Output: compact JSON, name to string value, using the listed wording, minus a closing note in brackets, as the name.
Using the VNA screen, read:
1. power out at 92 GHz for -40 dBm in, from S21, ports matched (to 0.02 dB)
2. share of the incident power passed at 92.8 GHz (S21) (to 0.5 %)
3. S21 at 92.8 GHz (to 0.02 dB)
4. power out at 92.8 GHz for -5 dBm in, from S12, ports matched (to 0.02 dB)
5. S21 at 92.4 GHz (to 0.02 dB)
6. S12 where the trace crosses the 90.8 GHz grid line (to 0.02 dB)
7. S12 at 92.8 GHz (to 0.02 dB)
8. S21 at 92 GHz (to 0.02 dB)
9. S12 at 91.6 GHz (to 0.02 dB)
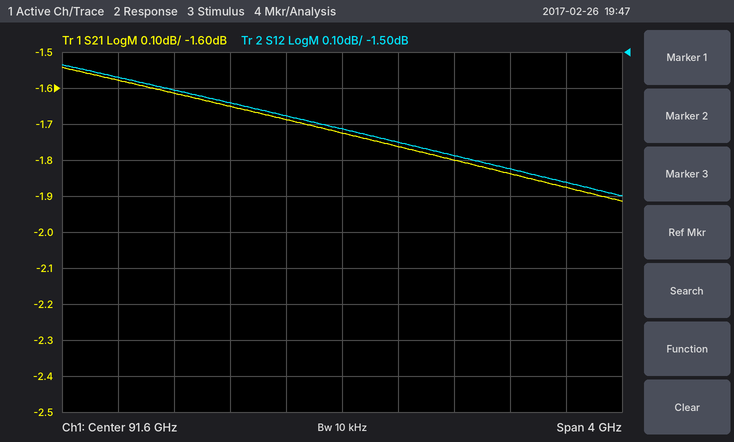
{"power out at 92 GHz for -40 dBm in, from S21, ports matched": "-41.76 dBm", "share of the incident power passed at 92.8 GHz (S21)": "65.5 %", "S21 at 92.8 GHz": "-1.84 dB", "power out at 92.8 GHz for -5 dBm in, from S12, ports matched": "-6.82 dBm", "S21 at 92.4 GHz": "-1.80 dB", "S12 where the trace crosses the 90.8 GHz grid line": "-1.64 dB", "S12 at 92.8 GHz": "-1.82 dB", "S21 at 92 GHz": "-1.76 dB", "S12 at 91.6 GHz": "-1.72 dB"}
